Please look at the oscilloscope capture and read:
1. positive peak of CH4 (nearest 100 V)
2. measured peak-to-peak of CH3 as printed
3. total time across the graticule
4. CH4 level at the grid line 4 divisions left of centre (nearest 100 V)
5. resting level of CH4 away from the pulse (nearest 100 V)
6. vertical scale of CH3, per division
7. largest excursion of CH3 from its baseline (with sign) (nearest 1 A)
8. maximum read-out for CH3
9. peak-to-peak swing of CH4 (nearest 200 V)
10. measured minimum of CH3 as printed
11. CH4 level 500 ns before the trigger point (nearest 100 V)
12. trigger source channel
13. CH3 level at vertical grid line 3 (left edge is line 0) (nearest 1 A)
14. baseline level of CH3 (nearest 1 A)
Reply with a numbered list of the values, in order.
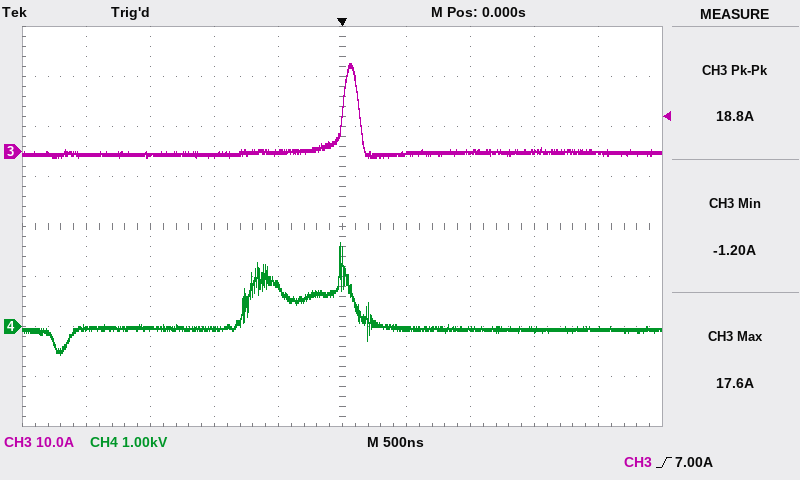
1. 1.7 kV
2. 18.8 A
3. 5 µs
4. 0.0 kV
5. -100 V
6. 10 A
7. +18 A
8. 17.6 A
9. 2.2 kV
10. -1.20 A
11. 800 V
12. CH3
13. -1 A
14. 0 A
